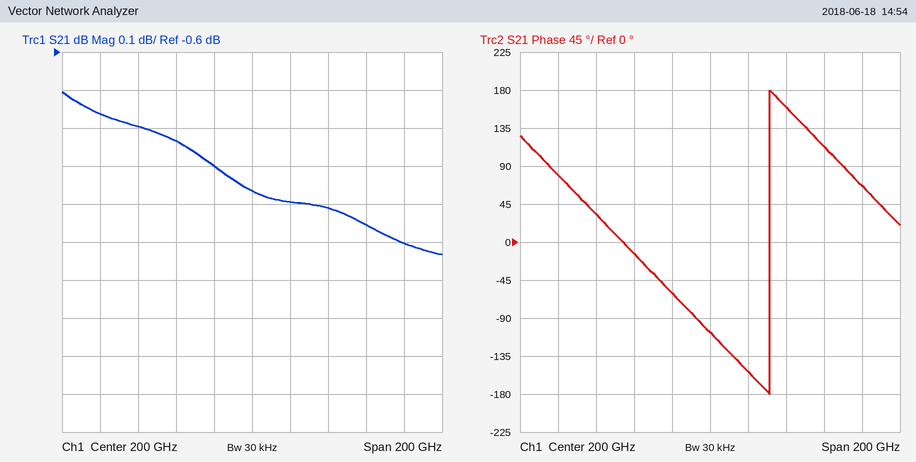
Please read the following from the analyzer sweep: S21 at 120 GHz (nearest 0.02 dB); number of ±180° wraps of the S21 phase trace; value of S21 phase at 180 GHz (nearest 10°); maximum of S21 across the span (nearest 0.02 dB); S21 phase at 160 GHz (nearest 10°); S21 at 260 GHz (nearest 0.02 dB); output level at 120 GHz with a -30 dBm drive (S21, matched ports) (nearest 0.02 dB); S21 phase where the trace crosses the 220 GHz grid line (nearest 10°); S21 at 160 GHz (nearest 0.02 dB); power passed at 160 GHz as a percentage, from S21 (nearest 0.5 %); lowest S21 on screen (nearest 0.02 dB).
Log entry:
-0.76 dB
1
-60°
-0.70 dB
-10°
-1.06 dB
-30.76 dBm
-150°
-0.84 dB
82.5 %
-1.14 dB
